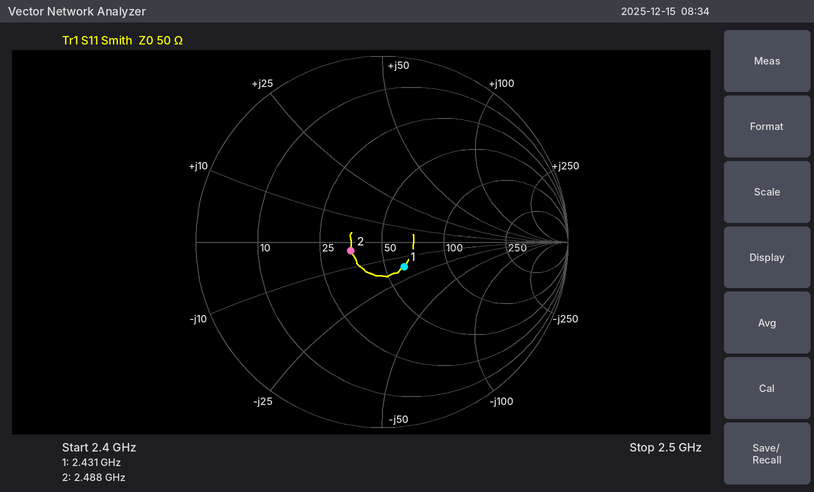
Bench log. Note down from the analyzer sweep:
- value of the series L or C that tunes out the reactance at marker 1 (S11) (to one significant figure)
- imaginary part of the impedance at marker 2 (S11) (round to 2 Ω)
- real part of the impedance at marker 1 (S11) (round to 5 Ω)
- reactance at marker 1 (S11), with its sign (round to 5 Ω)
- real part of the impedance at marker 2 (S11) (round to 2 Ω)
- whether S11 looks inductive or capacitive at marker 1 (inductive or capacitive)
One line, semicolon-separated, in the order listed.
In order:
1 nH; -4 Ω; 60 Ω; -15 Ω; 36 Ω; capacitive
